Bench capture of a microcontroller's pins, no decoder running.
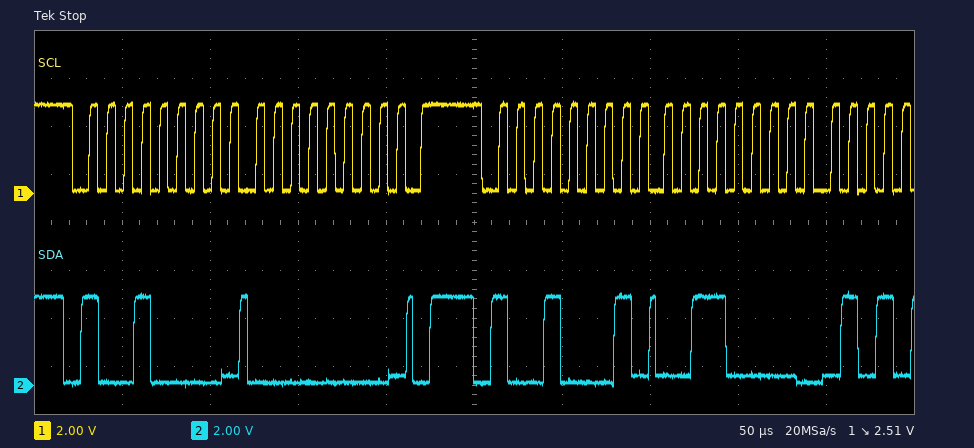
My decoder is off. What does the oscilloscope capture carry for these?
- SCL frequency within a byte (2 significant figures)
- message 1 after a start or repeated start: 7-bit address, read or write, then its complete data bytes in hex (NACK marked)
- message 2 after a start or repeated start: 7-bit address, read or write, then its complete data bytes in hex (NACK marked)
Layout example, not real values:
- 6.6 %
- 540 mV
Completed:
- 100 kHz
- 0x48 write: 00
- 0x48 read: 30
